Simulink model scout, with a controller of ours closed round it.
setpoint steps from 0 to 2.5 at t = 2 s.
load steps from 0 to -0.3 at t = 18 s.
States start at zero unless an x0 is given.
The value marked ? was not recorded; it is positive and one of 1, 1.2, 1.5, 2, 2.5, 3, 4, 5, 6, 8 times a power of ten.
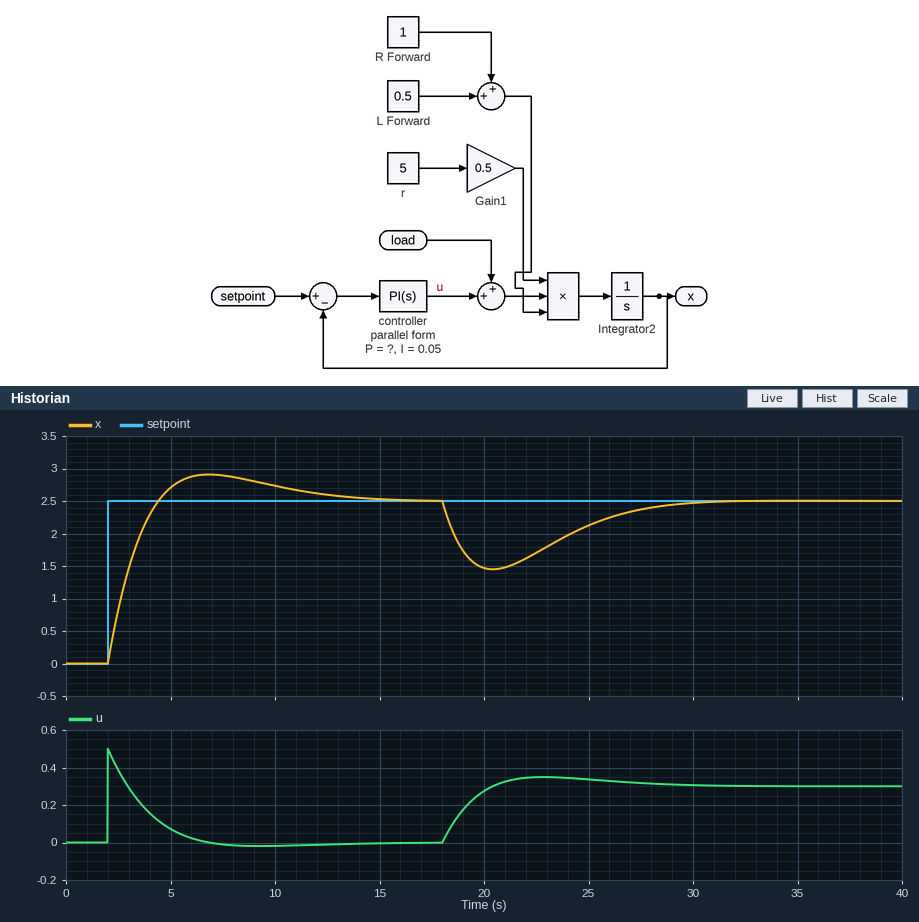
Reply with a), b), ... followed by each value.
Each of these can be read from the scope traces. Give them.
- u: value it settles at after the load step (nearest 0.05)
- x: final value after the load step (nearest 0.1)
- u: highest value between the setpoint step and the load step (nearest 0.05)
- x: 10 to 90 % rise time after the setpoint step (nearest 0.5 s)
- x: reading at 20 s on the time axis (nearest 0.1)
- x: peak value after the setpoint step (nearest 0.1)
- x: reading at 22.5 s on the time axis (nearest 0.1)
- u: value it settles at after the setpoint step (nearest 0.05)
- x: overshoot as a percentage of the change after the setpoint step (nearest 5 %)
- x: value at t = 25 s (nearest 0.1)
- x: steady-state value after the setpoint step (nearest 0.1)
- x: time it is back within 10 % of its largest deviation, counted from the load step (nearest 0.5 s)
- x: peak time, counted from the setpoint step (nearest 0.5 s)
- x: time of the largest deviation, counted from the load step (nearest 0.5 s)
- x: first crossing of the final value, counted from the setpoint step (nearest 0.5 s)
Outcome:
a) 0.30
b) 2.5
c) 0.50
d) 2.0 s
e) 1.5
f) 2.9
g) 1.7
h) 0.00
i) 15 %
j) 2.1
k) 2.5
l) 10.0 s
m) 5.0 s
n) 2.5 s
o) 2.5 s
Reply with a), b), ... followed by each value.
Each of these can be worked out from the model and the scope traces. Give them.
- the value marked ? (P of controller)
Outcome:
a) 0.2
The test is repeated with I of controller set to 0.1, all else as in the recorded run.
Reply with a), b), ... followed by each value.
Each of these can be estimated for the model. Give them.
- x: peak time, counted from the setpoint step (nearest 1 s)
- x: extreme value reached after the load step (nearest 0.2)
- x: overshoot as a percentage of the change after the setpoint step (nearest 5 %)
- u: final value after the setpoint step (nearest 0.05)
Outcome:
a) 4 s
b) 1.6
c) 25 %
d) 0.00
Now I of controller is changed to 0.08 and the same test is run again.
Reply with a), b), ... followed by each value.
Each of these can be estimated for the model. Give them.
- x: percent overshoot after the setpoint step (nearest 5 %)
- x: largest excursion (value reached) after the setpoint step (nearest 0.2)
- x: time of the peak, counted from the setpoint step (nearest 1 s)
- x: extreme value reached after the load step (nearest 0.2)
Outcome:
a) 20 %
b) 3.0
c) 4 s
d) 1.6
